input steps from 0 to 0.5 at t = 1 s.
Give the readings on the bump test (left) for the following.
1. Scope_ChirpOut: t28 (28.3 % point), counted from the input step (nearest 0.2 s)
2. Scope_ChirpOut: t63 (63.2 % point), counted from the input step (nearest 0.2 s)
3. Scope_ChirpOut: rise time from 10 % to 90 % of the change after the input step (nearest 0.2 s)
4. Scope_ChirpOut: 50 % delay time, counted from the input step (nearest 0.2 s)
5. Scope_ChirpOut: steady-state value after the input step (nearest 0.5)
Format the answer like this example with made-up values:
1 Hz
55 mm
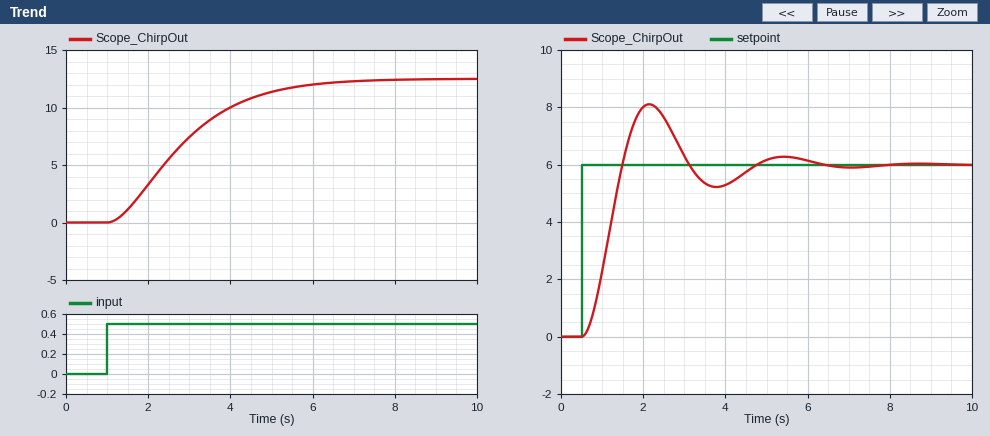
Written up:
1.0 s
2.2 s
3.4 s
1.6 s
12.5
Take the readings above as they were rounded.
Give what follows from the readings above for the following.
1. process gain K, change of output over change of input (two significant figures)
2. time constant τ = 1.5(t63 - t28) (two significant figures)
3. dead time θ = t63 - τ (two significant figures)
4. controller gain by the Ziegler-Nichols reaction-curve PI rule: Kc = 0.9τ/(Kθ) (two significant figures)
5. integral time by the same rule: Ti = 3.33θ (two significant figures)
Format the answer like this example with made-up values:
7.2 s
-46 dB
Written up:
25
1.8 s
0.40 s
0.16
1.3 s
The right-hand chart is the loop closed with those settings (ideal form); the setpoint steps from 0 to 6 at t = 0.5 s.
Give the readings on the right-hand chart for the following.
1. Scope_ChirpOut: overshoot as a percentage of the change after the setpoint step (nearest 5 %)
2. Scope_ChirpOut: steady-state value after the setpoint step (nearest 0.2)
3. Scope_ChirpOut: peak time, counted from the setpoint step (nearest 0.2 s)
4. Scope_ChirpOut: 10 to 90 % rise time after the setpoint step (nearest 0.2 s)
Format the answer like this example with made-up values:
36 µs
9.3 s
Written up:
35 %
6.0
1.6 s
0.6 s
